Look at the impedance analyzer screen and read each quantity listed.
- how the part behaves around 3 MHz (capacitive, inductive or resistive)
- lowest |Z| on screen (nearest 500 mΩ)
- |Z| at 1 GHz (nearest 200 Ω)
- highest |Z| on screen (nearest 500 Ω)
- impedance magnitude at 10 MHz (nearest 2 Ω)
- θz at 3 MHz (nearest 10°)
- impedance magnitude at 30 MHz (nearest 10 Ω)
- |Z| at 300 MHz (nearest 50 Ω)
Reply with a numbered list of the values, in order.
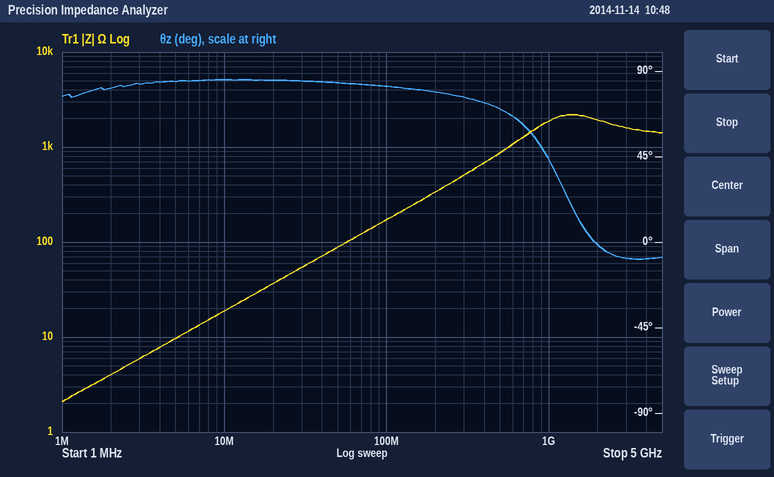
1. inductive
2. 2.0 Ω
3. 1.8 kΩ
4. 2.0 kΩ
5. 18 Ω
6. 80°
7. 50 Ω
8. 500 Ω
